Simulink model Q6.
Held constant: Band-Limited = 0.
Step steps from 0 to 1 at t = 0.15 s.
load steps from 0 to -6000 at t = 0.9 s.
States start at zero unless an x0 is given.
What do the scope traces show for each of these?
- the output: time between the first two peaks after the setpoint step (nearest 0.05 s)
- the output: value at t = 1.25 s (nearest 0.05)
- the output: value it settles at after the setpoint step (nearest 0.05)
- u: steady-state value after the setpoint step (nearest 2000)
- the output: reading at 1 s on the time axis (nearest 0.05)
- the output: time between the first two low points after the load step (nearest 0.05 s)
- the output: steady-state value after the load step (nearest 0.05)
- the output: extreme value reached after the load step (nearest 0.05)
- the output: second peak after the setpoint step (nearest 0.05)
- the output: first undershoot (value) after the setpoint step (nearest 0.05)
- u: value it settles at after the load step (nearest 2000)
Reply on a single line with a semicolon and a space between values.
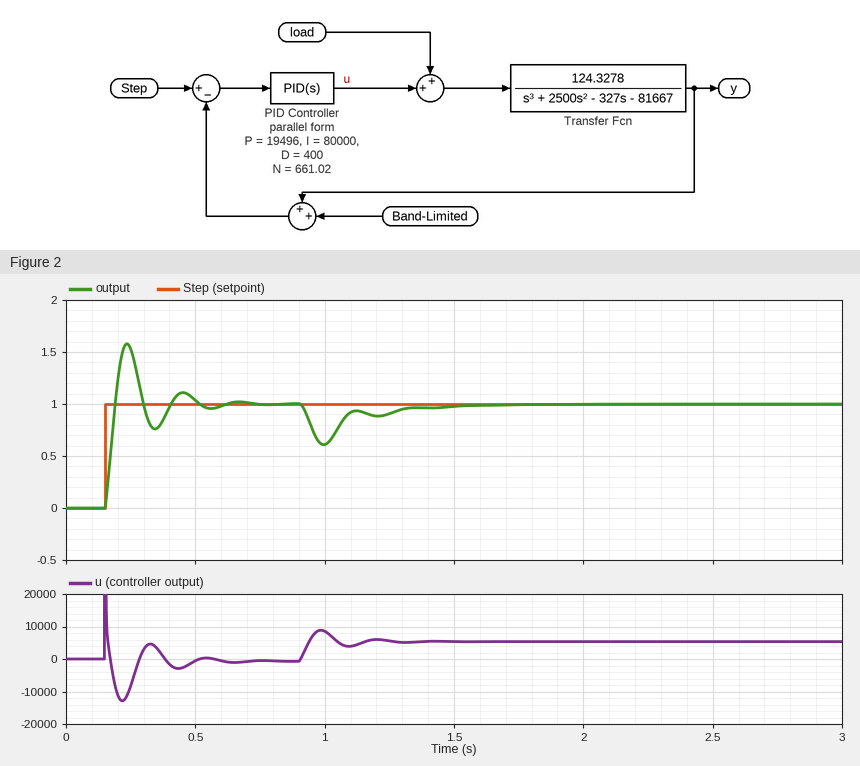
0.20 s; 0.90; 1.00; 0; 0.60; 0.20 s; 1.00; 0.60; 1.10; 0.75; 6000
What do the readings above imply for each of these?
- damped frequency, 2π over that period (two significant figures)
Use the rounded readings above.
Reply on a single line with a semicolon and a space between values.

31 rad/s
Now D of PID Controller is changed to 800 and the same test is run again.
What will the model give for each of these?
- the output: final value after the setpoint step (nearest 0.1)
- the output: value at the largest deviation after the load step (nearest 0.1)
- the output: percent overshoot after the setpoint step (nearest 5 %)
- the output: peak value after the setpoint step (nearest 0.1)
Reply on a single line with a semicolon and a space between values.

1.0; 0.7; 30 %; 1.3
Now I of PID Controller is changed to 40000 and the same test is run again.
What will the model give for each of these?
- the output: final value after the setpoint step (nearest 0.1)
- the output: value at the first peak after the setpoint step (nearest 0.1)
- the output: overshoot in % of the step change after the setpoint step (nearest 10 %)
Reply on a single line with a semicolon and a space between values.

1.0; 1.5; 50 %
